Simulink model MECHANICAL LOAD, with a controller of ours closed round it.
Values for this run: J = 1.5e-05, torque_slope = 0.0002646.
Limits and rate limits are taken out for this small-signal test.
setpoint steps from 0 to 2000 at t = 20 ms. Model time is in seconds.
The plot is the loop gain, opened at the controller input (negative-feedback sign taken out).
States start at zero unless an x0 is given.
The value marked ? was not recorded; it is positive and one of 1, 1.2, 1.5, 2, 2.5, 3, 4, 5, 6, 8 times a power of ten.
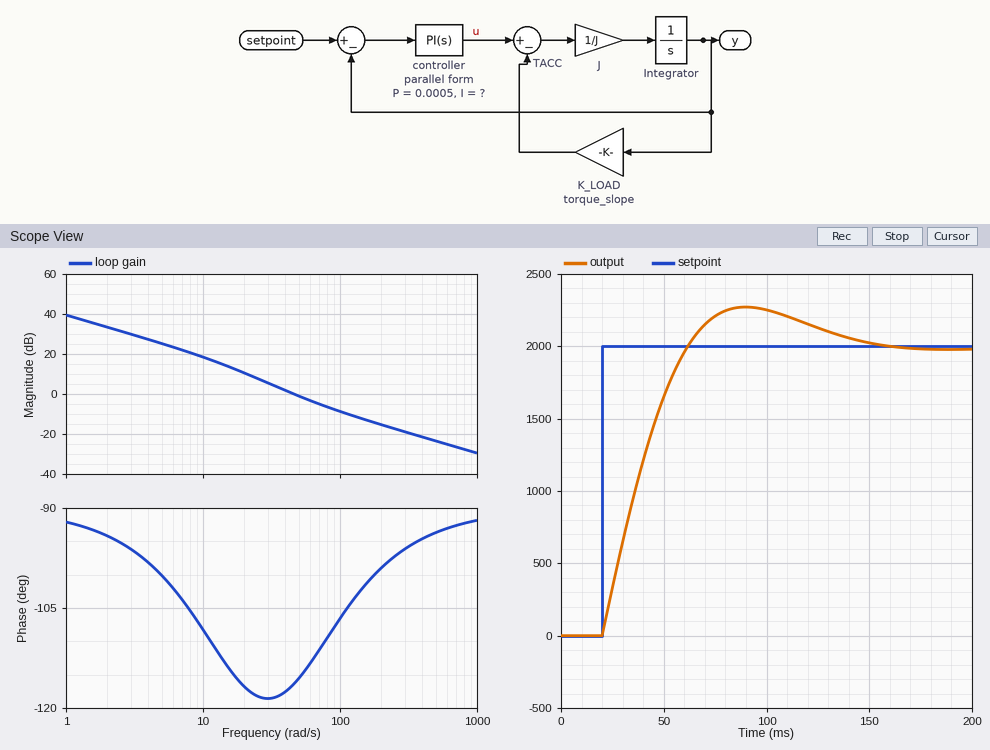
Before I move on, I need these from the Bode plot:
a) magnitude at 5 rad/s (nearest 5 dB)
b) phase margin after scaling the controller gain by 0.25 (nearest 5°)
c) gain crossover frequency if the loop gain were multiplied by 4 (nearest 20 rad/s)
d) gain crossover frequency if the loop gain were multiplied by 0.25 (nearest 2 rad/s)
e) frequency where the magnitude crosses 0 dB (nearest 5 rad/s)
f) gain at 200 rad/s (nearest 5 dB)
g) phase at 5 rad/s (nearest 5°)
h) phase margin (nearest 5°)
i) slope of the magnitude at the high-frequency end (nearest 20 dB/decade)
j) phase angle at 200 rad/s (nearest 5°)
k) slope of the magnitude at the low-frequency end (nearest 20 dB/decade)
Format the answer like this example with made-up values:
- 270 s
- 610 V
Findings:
- 25 dB
- 65°
- 140 rad/s
- 18 rad/s
- 45 rad/s
- -15 dB
- -100°
- 65°
- -20 dB/decade
- -100°
- -20 dB/decade
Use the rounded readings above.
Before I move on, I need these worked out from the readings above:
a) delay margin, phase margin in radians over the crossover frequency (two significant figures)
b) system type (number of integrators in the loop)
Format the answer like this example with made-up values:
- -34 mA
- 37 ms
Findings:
- 0.025 s
- 1
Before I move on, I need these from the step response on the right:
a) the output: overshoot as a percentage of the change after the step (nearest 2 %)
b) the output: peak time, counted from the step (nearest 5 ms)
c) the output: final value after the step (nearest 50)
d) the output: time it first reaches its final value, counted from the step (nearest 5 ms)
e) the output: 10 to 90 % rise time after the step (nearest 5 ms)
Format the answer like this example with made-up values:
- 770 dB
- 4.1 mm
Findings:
- 14 %
- 70 ms
- 2000
- 40 ms
- 30 ms
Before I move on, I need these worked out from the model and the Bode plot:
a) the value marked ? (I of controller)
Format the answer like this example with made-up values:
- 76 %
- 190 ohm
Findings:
- 0.025
